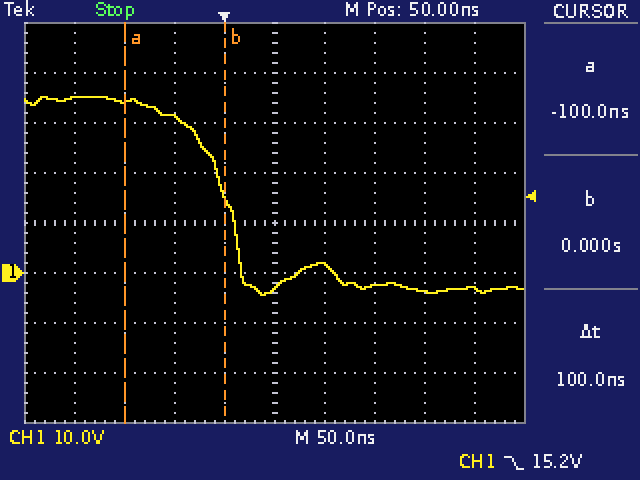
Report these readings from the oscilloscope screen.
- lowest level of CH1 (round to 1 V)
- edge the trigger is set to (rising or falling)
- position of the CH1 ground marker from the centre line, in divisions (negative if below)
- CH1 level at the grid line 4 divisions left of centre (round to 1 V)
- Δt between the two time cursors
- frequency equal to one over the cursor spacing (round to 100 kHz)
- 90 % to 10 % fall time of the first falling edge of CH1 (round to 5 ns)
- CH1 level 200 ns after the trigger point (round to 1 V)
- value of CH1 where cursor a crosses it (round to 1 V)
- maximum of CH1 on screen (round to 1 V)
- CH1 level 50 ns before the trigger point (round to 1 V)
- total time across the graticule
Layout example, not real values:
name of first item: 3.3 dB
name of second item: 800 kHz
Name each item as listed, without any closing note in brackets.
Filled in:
lowest level of CH1: -4 V
edge the trigger is set to: falling
position of the CH1 ground marker from the centre line, in divisions: -1.0 div
CH1 level at the grid line 4 divisions left of centre: 35 V
Δt between the two time cursors: 100 ns
frequency equal to one over the cursor spacing: 10.0 MHz
90 % to 10 % fall time of the first falling edge of CH1: 65 ns
CH1 level 200 ns after the trigger point: -4 V
value of CH1 where cursor a crosses it: 34 V
maximum of CH1 on screen: 35 V
CH1 level 50 ns before the trigger point: 31 V
total time across the graticule: 500 ns
